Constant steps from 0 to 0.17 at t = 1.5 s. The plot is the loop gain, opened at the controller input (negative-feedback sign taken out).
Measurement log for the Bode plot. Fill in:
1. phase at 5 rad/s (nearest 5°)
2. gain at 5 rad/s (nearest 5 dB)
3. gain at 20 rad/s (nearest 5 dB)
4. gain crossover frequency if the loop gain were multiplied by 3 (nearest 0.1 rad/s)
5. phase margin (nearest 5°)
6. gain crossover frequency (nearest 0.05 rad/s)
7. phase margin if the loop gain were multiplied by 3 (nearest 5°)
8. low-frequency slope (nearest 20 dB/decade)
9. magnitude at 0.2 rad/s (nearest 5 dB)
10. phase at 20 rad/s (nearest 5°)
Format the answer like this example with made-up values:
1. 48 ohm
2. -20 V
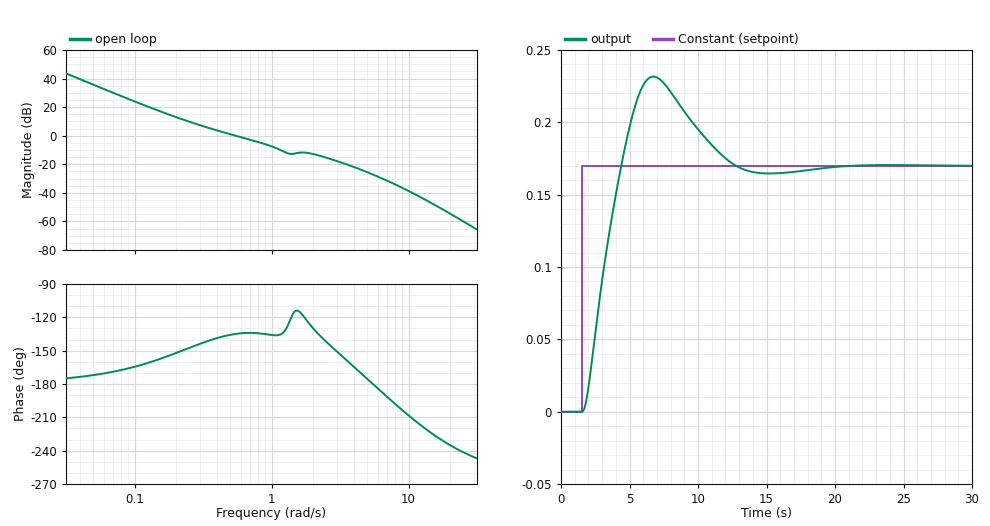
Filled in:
1. -175°
2. -25 dB
3. -55 dB
4. 1.1 rad/s
5. 45°
6. 0.55 rad/s
7. 45°
8. -40 dB/decade
9. 15 dB
10. -235°
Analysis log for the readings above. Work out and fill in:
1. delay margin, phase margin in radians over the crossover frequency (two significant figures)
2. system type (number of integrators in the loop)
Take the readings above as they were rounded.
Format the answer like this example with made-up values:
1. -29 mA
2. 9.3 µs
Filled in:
1. 1.4 s
2. 2
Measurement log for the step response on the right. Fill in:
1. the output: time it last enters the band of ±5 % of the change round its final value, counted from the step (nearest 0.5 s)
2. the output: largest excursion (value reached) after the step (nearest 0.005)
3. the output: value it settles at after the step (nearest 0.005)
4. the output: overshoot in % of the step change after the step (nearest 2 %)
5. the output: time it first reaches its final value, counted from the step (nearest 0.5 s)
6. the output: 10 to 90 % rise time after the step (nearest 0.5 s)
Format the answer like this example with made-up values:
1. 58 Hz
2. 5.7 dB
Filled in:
1. 10.0 s
2. 0.230
3. 0.170
4. 36 %
5. 3.0 s
6. 2.0 s
